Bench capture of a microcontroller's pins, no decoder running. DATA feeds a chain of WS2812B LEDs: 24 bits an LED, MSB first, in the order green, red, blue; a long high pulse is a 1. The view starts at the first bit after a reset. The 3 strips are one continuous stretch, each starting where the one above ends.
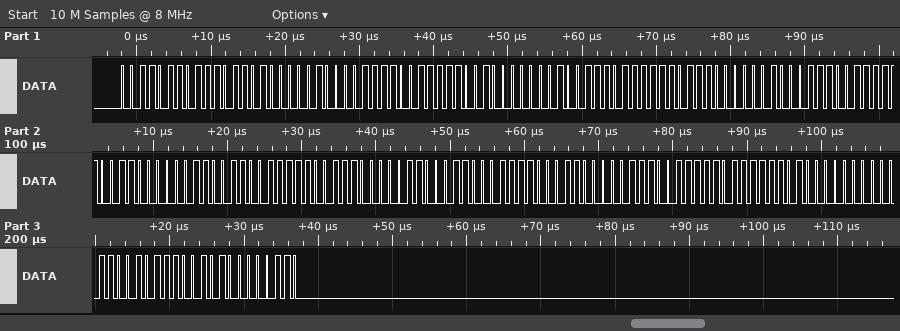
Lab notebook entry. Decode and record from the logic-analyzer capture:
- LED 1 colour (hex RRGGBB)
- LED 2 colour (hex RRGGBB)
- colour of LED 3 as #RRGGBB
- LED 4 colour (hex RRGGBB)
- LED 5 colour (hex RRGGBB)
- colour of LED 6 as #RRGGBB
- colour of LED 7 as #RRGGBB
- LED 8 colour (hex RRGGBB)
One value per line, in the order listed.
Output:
#ED3604
#F93C01
#F73B02
#F33903
#E73306
#E33107
#FD3E00
#E53206
